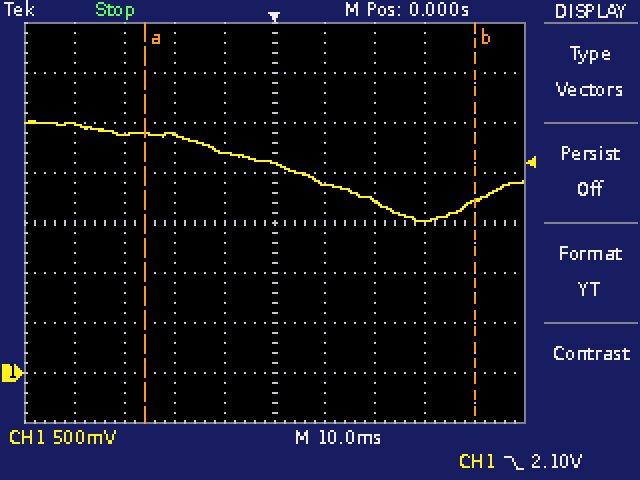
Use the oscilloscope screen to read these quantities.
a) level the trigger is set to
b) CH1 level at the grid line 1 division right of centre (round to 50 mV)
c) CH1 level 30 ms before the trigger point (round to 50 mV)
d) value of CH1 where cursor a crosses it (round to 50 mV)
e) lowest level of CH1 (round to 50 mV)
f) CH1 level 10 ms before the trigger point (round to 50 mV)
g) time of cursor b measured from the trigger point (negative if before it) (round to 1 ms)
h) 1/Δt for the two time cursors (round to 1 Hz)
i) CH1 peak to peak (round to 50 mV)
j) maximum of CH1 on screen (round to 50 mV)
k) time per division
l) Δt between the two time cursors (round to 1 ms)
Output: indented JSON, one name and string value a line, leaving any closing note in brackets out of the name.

{
  "level the trigger is set to": "2.10 V",
  "CH1 level at the grid line 1 division right of centre": "1.90 V",
  "CH1 level 30 ms before the trigger point": "2.40 V",
  "value of CH1 where cursor a crosses it": "2.40 V",
  "lowest level of CH1": "1.50 V",
  "CH1 level 10 ms before the trigger point": "2.20 V",
  "time of cursor b measured from the trigger point (negative if before it)": "+40 ms",
  "1/Δt for the two time cursors": "15 Hz",
  "CH1 peak to peak": "1.00 V",
  "maximum of CH1 on screen": "2.50 V",
  "time per division": "10 ms",
  "Δt between the two time cursors": "66 ms"
}
